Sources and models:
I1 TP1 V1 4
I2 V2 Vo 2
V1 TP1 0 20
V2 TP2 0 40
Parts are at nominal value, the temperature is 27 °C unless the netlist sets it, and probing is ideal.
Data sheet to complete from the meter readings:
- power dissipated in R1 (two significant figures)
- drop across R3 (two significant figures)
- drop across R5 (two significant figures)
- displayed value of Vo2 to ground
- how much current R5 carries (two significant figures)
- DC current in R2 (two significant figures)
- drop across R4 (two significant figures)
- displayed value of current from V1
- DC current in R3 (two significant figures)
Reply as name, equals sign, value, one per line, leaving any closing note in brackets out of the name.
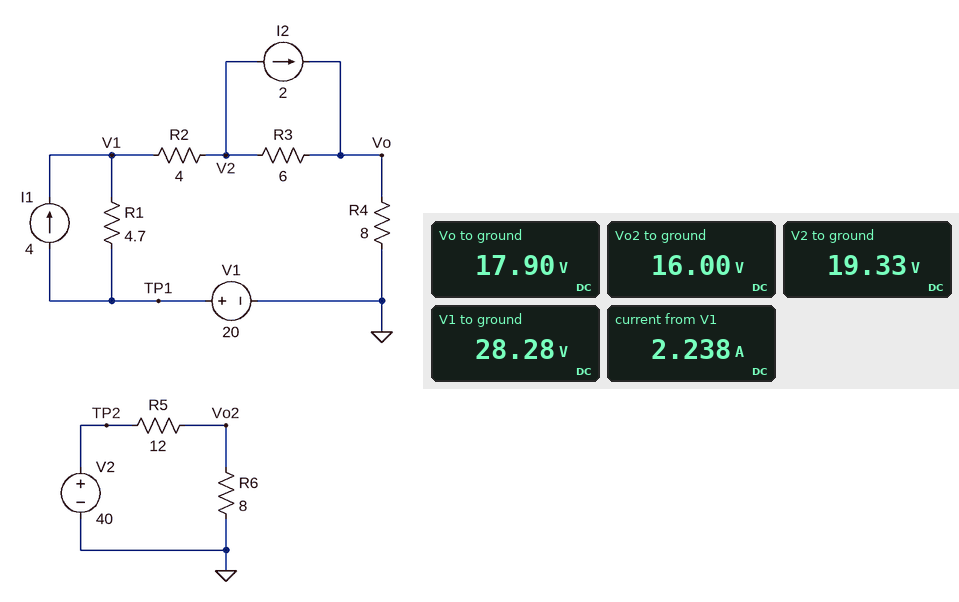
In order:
power dissipated in R1 = 15 W
drop across R3 = 1.4 V
drop across R5 = 24 V
displayed value of Vo2 to ground = 16.00 V
how much current R5 carries = 2.0 A
DC current in R2 = 2.2 A
drop across R4 = 18 V
displayed value of current from V1 = 2.238 A
DC current in R3 = 240 mA
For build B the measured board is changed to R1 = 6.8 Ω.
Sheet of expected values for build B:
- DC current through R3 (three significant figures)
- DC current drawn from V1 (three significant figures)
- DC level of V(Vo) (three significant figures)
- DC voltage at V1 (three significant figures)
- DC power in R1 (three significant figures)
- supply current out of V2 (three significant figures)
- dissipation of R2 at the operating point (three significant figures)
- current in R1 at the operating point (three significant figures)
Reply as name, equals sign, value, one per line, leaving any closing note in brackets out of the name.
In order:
DC current through R3 = 387 mA
DC current drawn from V1 = 2.39 A
DC level of V(Vo) = 19.1 V
DC voltage at V1 = 31.0 V
DC power in R1 = 17.7 W
supply current out of V2 = 2.00 A
dissipation of R2 at the operating point = 22.8 W
current in R1 at the operating point = 1.61 A
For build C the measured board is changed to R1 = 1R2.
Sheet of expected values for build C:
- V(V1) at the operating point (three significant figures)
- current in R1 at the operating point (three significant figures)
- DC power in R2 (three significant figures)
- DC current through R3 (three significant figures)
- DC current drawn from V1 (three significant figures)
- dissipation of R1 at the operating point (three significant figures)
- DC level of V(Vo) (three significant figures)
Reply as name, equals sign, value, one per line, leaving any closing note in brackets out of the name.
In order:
V(V1) at the operating point = 22.5 V
current in R1 at the operating point = 2.08 A
DC power in R2 = 14.7 W
DC current through R3 = 83.3 mA
DC current drawn from V1 = 1.92 A
dissipation of R1 at the operating point = 5.21 W
DC level of V(Vo) = 15.3 V
